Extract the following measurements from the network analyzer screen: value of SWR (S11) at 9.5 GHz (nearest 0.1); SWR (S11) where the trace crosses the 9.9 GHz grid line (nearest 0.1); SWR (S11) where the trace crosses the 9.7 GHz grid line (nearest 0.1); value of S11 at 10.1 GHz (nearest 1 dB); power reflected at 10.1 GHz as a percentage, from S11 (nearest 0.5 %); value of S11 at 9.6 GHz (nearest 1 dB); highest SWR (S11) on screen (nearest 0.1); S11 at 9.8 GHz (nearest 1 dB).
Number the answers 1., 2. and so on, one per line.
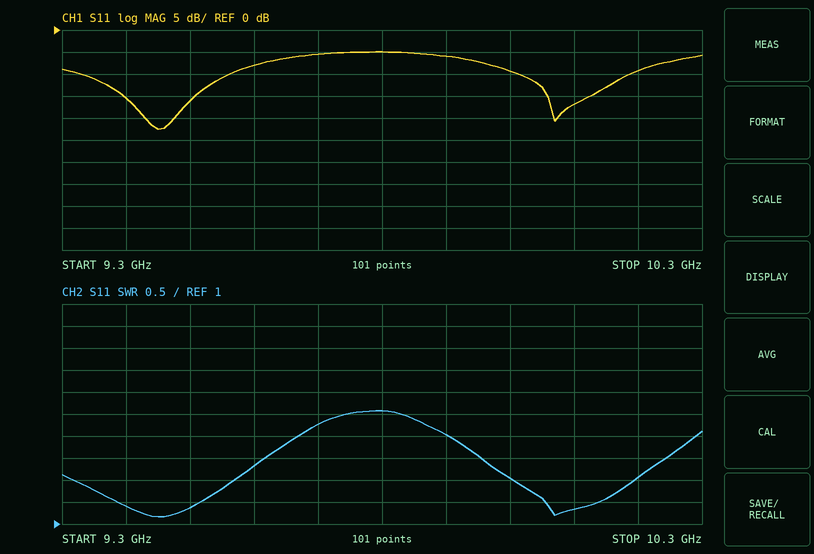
1. 1.4
2. 3.0
3. 3.3
4. -17 dB
5. 2.0 %
6. -8 dB
7. 3.6
8. -5 dB
